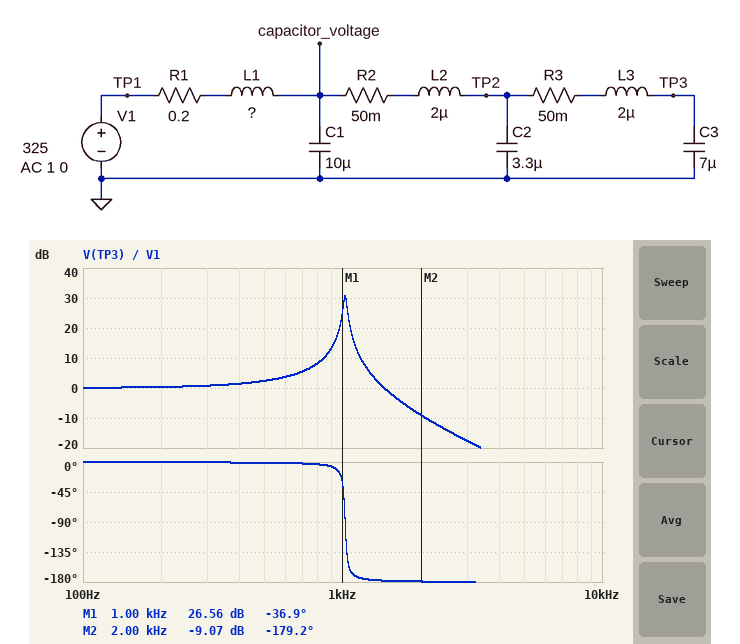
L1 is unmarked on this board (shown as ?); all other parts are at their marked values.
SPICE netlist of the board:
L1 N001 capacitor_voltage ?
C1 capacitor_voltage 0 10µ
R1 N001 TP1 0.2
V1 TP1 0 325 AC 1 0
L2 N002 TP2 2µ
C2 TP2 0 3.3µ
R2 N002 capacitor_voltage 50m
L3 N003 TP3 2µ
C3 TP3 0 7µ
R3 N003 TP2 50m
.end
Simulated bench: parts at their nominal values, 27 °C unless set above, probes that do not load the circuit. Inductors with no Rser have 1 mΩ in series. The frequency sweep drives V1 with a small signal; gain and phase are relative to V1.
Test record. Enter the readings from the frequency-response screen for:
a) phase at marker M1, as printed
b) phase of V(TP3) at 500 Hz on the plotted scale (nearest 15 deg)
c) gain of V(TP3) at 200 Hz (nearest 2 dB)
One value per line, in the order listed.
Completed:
-36.9 deg
0 deg
0 dB
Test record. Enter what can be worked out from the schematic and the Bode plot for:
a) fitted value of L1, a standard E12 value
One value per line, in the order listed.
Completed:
1.2 mH
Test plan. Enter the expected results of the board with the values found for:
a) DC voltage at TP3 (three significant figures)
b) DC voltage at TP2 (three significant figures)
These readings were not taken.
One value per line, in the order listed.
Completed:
325 V
325 V
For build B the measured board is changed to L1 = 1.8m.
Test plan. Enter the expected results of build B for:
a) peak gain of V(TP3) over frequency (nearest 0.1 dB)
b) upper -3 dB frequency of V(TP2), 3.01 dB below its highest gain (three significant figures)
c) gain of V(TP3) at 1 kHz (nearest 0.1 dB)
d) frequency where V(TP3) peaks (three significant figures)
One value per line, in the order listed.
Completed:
32.6 dB
842 Hz
7.1 dB
832 Hz
